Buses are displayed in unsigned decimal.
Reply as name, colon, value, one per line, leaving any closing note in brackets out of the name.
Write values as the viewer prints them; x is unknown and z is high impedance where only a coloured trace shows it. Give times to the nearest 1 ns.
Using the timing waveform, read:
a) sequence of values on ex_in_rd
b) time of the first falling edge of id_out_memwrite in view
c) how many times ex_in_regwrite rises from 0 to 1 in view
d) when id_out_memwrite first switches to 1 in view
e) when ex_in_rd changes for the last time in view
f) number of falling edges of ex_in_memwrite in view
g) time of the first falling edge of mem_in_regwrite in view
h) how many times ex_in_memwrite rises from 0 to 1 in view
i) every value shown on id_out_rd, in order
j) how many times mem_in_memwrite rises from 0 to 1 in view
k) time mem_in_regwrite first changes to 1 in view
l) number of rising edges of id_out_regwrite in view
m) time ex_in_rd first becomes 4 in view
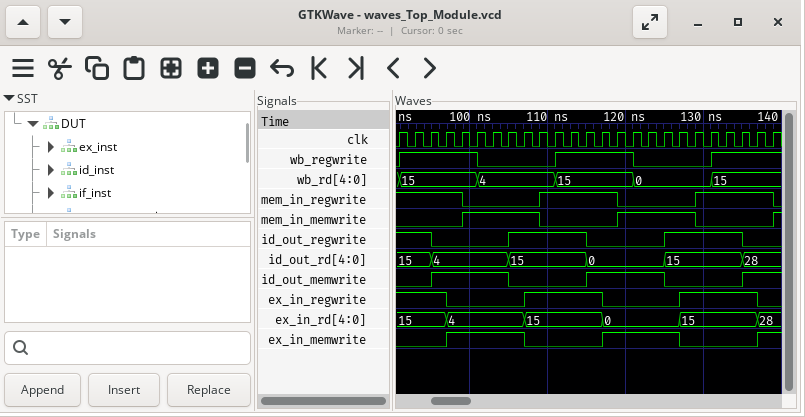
sequence of values on ex_in_rd: 15, 4, 15, 0, 15, 28
time of the first falling edge of id_out_memwrite in view: 105 ns
how many times ex_in_regwrite rises from 0 to 1 in view: 2
when id_out_memwrite first switches to 1 in view: 95 ns
when ex_in_rd changes for the last time in view: 137 ns
number of falling edges of ex_in_memwrite in view: 2
time of the first falling edge of mem_in_regwrite in view: 99 ns
how many times ex_in_memwrite rises from 0 to 1 in view: 3
every value shown on id_out_rd, in order: 15, 4, 15, 0, 15, 28
how many times mem_in_memwrite rises from 0 to 1 in view: 3
time mem_in_regwrite first changes to 1 in view: 109 ns
number of rising edges of id_out_regwrite in view: 2
time ex_in_rd first becomes 4 in view: 97 ns
